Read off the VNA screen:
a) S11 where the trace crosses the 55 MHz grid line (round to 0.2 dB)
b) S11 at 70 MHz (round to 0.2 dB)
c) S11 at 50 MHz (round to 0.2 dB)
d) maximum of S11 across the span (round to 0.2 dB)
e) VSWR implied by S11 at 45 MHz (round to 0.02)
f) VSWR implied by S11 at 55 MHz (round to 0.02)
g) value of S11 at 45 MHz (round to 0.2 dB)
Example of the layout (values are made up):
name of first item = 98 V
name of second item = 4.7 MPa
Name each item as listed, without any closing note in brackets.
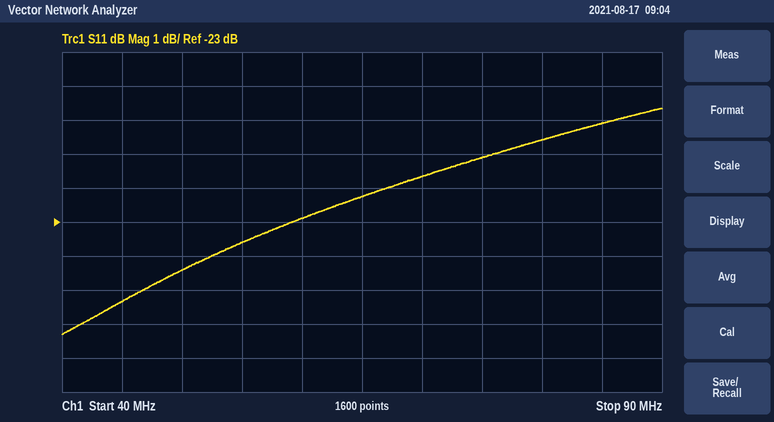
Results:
S11 where the trace crosses the 55 MHz grid line = -23.6 dB
S11 at 70 MHz = -21.6 dB
S11 at 50 MHz = -24.4 dB
maximum of S11 across the span = -19.6 dB
VSWR implied by S11 at 45 MHz = 1.12
VSWR implied by S11 at 55 MHz = 1.14
value of S11 at 45 MHz = -25.4 dB
